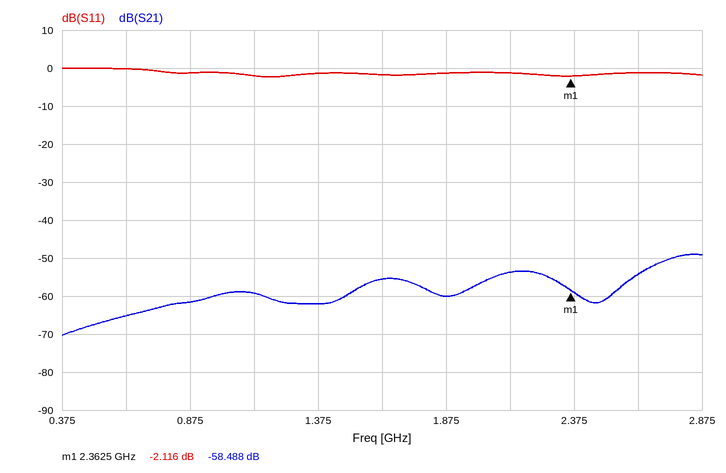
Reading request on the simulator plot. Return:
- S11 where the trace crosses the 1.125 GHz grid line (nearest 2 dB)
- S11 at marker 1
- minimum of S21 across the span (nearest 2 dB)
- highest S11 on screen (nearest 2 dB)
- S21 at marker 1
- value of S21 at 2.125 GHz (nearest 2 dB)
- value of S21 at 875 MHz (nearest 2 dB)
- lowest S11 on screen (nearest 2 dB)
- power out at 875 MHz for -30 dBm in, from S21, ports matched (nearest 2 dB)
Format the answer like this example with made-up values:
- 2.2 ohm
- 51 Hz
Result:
- -2 dB
- -2.116 dB
- -70 dB
- 0 dB
- -58.488 dB
- -54 dB
- -62 dB
- -2 dB
- -92 dBm
